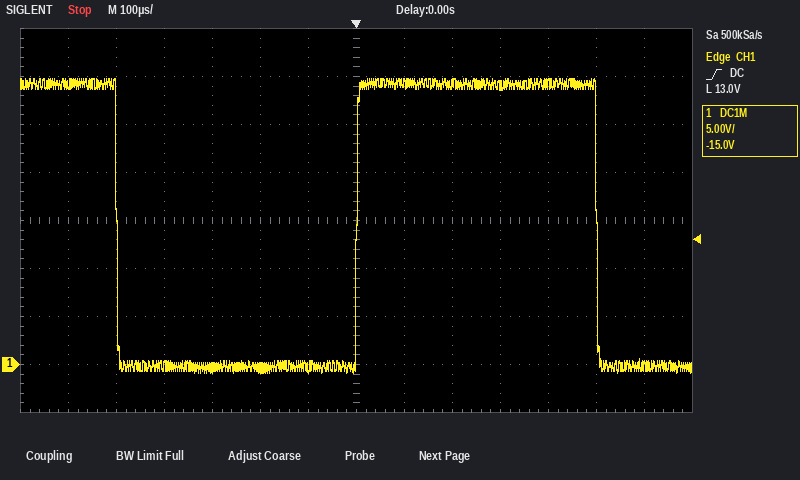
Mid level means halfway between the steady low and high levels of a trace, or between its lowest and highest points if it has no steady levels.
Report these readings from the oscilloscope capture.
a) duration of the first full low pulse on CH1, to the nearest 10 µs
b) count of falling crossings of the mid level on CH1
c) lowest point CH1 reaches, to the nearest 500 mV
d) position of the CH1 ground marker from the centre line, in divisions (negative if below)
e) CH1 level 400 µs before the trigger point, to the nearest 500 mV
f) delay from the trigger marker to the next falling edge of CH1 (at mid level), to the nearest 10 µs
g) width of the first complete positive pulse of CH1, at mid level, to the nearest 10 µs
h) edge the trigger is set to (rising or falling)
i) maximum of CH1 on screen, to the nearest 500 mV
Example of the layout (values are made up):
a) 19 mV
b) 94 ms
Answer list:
a) 500 µs
b) 2
c) -1.0 V
d) -3.0 div
e) 0.0 V
f) 500 µs
g) 500 µs
h) rising
i) 30.0 V
